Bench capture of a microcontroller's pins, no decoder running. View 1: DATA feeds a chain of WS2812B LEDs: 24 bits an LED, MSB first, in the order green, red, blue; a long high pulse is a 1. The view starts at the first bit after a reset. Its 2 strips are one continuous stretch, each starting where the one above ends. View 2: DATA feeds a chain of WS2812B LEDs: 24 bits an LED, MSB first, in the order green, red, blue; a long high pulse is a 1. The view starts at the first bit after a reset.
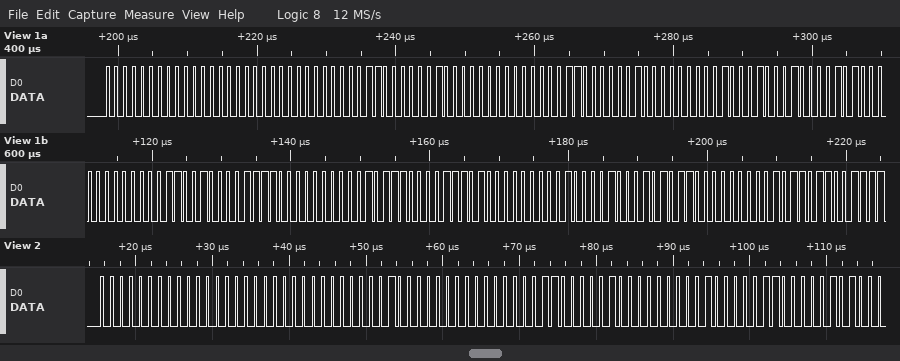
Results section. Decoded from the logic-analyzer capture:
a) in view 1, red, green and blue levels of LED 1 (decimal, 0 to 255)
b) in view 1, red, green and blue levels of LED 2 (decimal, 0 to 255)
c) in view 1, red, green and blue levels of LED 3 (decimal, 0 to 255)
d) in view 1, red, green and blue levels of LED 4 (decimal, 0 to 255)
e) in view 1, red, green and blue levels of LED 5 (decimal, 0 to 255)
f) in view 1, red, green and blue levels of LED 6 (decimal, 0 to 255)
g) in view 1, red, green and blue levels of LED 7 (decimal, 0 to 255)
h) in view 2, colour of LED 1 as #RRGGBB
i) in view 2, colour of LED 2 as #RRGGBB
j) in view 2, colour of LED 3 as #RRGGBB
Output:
0, 0, 0
2, 3, 0
4, 6, 1
10, 17, 0
15, 25, 0
29, 46, 0
43, 66, 0
#000000
#000203
#010406
